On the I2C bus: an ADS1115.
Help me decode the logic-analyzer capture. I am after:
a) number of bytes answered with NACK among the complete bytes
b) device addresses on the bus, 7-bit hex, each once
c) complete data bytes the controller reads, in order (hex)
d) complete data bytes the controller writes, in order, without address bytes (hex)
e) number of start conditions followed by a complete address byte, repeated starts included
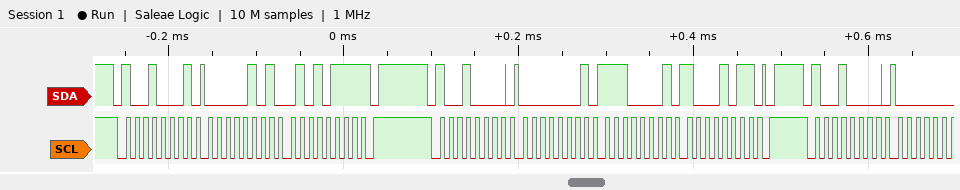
1
0x48
05 57
01 E1 8B
3
